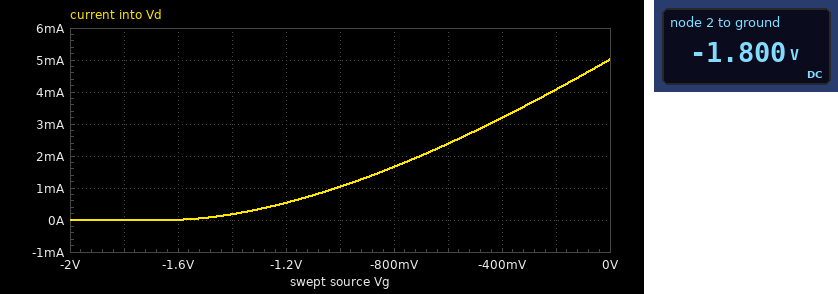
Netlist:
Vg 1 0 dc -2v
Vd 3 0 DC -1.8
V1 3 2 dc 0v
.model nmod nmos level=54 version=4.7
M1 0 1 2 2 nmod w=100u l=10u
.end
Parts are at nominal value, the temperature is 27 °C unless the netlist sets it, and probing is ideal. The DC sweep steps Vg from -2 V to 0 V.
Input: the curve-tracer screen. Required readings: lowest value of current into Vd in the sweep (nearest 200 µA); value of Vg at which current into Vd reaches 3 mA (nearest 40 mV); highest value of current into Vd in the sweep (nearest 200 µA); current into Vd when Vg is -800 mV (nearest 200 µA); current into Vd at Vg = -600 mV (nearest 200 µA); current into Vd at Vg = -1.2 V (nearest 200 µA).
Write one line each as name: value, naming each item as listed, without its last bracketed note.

lowest value of current into Vd in the sweep: 0 A
value of Vg at which current into Vd reaches 3 mA: -440 mV
highest value of current into Vd in the sweep: 5.0 mA
current into Vd when Vg is -800 mV: 1.6 mA
current into Vd at Vg = -600 mV: 2.4 mA
current into Vd at Vg = -1.2 V: 600 µA
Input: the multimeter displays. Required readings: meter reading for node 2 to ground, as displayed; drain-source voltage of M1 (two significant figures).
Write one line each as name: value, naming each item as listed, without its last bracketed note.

meter reading for node 2 to ground, as displayed: -1.800 V
drain-source voltage of M1: 1.8 V
